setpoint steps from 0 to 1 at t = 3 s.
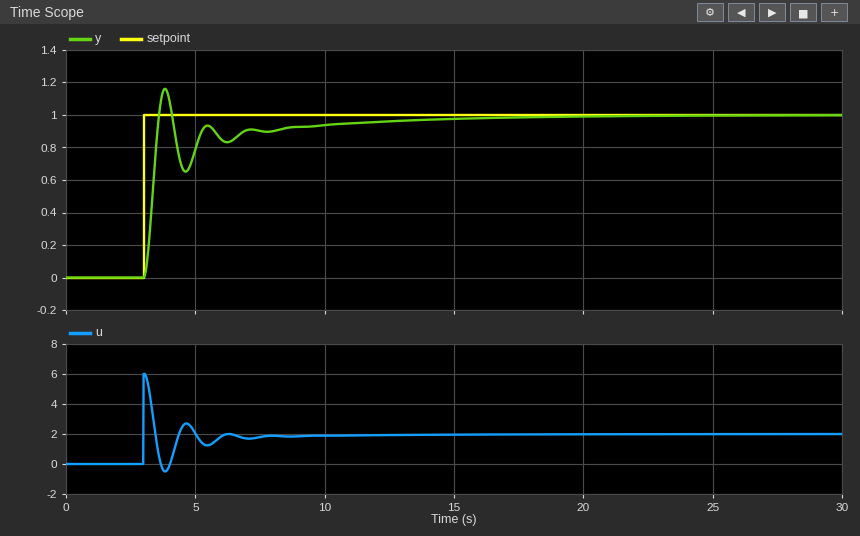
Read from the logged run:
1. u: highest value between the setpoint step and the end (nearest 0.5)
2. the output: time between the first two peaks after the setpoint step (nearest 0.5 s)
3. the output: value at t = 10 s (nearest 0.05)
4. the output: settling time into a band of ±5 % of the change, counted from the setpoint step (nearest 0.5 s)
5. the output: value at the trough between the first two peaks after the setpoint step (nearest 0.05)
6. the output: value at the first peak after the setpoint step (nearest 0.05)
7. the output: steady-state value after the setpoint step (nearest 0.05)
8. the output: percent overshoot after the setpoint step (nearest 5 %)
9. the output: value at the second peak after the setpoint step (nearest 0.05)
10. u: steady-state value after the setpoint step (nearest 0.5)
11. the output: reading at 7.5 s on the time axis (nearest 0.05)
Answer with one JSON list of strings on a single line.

["6.0", "1.5 s", "0.95", "8.0 s", "0.65", "1.15", "1.00", "15 %", "0.95", "2.0", "0.90"]
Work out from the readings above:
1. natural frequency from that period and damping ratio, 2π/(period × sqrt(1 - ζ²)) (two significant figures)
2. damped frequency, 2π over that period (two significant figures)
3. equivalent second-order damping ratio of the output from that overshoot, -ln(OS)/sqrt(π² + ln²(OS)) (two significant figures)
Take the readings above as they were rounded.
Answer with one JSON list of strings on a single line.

["4.9 rad/s", "4.2 rad/s", "0.52"]
